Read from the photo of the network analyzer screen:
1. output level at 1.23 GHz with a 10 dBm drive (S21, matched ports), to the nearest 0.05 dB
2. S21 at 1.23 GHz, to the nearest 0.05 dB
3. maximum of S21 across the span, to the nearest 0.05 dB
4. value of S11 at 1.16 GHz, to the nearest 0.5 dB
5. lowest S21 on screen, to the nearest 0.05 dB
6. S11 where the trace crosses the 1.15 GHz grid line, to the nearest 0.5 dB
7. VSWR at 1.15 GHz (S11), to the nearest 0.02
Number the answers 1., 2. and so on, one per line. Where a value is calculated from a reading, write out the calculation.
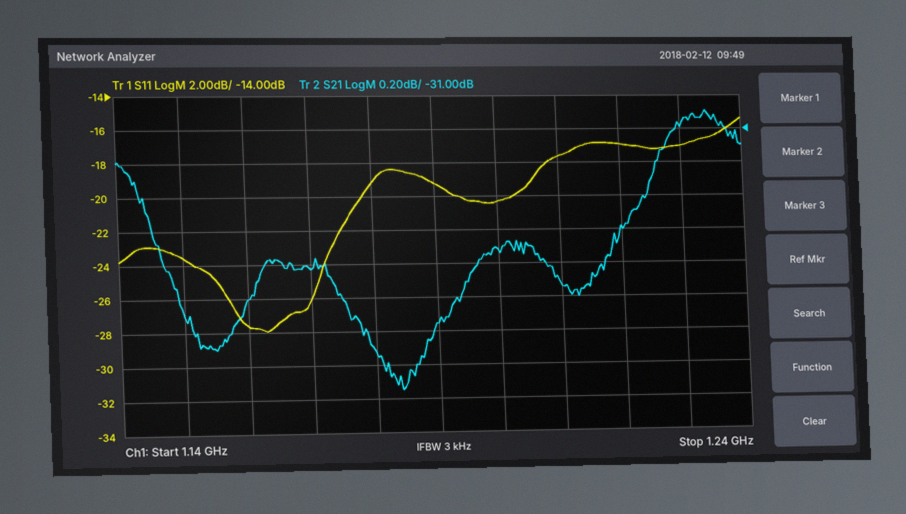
1. 10 dBm + (-31.00 dB) = -21.00 dBm
2. -31.00 dB
3. -30.90 dB
4. -27.5 dB
5. -32.55 dB
6. -23.5 dB
7. |Γ| = 10^(-23.5/20) = 0.0668; VSWR = (1 + 0.0668)/(1 − 0.0668) ≈ 1.14
